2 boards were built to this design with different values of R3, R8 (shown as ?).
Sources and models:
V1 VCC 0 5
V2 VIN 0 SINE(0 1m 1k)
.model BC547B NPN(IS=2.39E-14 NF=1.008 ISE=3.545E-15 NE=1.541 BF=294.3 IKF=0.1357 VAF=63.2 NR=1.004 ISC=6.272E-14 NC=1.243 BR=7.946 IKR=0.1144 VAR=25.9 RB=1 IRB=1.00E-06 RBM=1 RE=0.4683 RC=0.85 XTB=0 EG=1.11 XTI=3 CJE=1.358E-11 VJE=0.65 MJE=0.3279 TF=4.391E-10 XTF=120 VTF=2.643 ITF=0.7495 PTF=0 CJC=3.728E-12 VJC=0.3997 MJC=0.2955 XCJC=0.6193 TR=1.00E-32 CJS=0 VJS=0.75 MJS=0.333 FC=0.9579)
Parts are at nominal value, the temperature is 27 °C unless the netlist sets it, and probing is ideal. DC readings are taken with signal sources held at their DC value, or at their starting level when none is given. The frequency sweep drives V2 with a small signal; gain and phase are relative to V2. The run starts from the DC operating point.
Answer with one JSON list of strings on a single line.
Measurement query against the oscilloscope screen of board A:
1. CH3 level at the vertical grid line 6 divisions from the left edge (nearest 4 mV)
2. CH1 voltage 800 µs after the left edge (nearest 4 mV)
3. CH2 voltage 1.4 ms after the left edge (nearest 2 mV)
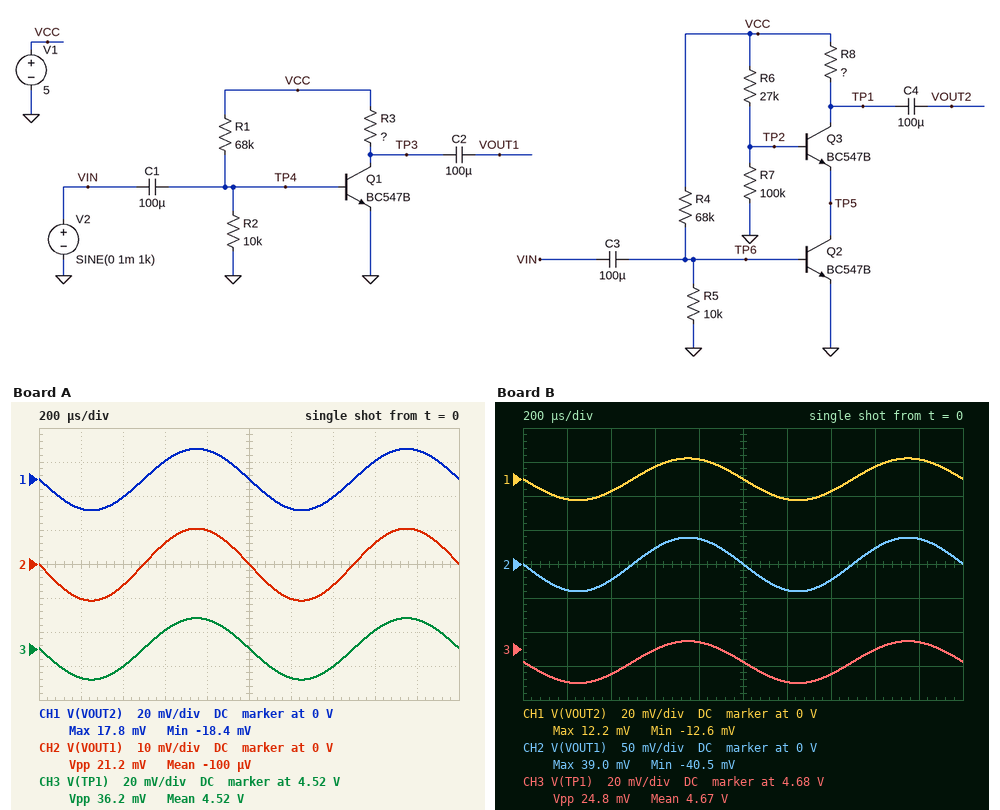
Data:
["4.504 V", "16 mV", "-6 mV"]
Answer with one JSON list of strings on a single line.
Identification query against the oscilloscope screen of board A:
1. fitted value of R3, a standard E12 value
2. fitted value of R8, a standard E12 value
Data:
["470 Ω", "820 Ω"]
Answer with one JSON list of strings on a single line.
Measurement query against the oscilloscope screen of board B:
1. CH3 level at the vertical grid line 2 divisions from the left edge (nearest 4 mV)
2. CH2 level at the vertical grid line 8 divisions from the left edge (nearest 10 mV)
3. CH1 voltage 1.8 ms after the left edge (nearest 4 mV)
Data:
["4.664 V", "20 mV", "12 mV"]
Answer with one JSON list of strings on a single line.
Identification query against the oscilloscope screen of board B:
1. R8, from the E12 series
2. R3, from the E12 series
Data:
["560 Ω", "1.8 kΩ"]
